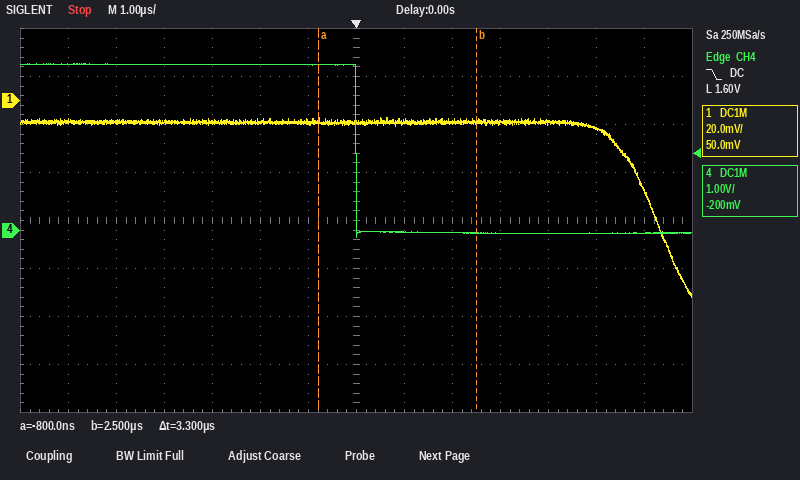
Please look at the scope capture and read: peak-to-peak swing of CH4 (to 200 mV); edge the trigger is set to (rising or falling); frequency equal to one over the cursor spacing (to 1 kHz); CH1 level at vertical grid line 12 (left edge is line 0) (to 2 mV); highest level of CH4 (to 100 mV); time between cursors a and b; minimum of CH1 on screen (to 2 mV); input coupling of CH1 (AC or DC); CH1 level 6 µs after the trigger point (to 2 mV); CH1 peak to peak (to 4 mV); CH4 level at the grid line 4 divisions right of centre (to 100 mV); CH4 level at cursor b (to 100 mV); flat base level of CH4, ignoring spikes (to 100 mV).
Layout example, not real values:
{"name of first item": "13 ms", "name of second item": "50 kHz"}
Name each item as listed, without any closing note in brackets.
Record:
{"peak-to-peak swing of CH4": "3.6 V", "edge the trigger is set to": "falling", "frequency equal to one over the cursor spacing": "303 kHz", "CH1 level at vertical grid line 12 (left edge is line 0)": "-12 mV", "highest level of CH4": "3.5 V", "time between cursors a and b": "3.3 µs", "minimum of CH1 on screen": "-82 mV", "input coupling of CH1": "DC", "CH1 level 6 µs after the trigger point": "-38 mV", "CH1 peak to peak": "76 mV", "CH4 level at the grid line 4 divisions right of centre": "-100 mV", "CH4 level at cursor b": "-100 mV", "flat base level of CH4, ignoring spikes": "-100 mV"}
